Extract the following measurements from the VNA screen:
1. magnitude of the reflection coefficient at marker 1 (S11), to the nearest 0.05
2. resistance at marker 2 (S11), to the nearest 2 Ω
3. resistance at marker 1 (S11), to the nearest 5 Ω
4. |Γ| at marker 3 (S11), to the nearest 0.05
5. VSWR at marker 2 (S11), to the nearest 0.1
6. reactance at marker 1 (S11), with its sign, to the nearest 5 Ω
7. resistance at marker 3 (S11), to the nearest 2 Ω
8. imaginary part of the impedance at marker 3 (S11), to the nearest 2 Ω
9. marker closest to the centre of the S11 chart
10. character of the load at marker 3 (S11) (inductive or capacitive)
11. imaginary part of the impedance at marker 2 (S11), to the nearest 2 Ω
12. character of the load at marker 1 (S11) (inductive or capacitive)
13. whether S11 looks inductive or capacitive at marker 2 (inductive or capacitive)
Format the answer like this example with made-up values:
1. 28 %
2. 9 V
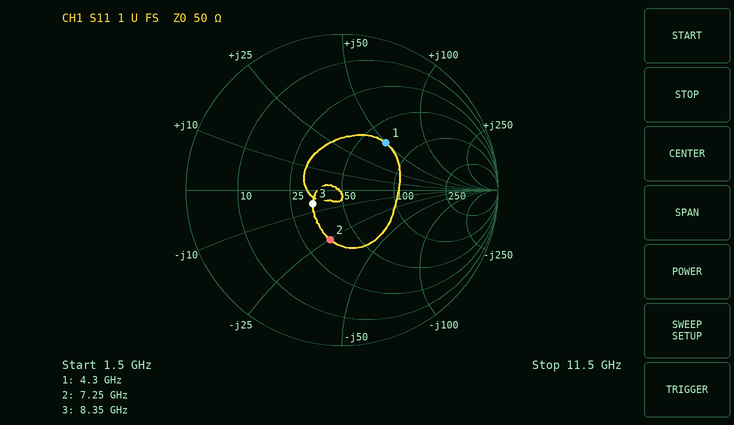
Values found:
1. 0.40
2. 36 Ω
3. 70 Ω
4. 0.20
5. 2.0
6. +50 Ω
7. 34 Ω
8. -6 Ω
9. marker 3
10. capacitive
11. -26 Ω
12. inductive
13. capacitive
